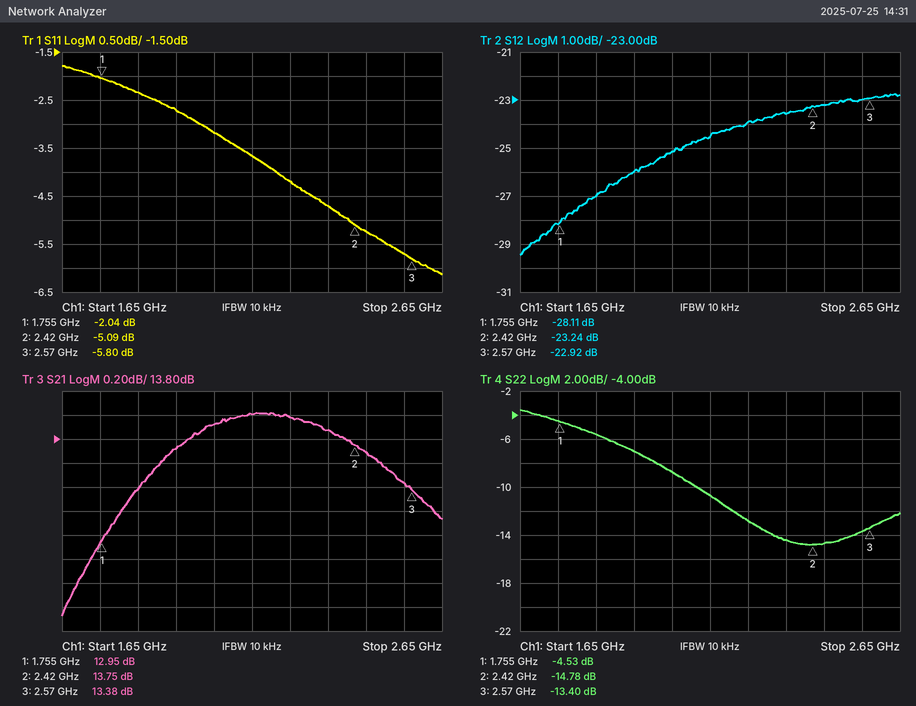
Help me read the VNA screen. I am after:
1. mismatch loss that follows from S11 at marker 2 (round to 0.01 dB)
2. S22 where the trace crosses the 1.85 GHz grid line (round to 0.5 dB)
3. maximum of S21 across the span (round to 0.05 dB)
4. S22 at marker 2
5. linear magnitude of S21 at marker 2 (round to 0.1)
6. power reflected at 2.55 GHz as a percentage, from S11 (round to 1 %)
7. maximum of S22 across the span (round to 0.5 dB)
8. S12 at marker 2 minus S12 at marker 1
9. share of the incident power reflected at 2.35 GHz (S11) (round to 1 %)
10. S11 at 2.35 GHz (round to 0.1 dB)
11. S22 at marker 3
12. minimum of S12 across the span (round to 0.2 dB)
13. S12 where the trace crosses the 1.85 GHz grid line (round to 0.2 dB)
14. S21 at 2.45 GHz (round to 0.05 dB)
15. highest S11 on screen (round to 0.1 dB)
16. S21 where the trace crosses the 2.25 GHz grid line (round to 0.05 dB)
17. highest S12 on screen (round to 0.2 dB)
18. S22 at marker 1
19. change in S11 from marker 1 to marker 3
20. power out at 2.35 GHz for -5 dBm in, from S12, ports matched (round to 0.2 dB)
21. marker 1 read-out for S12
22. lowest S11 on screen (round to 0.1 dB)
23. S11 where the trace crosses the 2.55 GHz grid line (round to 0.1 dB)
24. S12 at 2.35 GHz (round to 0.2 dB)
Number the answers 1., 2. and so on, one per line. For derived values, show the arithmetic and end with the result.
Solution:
1. −10 log10(1 − 10^(-5.09/10)) ≈ 1.61 dB
2. -5.5 dB
3. 14.00 dB
4. -14.78 dB
5. 10^(13.75/20) ≈ 4.9
6. 10^(-5.7/10) ≈ 27 %
7. -3.5 dB
8. -23.24 − (-28.11) = 4.87 dB
9. 10^(-4.7/10) ≈ 34 %
10. -4.7 dB
11. -13.40 dB
12. -29.4 dB
13. -27.0 dB
14. 13.70 dB
15. -1.8 dB
16. 14.00 dB
17. -22.8 dB
18. -4.53 dB
19. -5.8 − (-2.04) = -3.76 dB
20. -5 dBm + (-23.6 dB) = -28.6 dBm
21. -28.11 dB
22. -6.1 dB
23. -5.7 dB
24. -23.6 dB
